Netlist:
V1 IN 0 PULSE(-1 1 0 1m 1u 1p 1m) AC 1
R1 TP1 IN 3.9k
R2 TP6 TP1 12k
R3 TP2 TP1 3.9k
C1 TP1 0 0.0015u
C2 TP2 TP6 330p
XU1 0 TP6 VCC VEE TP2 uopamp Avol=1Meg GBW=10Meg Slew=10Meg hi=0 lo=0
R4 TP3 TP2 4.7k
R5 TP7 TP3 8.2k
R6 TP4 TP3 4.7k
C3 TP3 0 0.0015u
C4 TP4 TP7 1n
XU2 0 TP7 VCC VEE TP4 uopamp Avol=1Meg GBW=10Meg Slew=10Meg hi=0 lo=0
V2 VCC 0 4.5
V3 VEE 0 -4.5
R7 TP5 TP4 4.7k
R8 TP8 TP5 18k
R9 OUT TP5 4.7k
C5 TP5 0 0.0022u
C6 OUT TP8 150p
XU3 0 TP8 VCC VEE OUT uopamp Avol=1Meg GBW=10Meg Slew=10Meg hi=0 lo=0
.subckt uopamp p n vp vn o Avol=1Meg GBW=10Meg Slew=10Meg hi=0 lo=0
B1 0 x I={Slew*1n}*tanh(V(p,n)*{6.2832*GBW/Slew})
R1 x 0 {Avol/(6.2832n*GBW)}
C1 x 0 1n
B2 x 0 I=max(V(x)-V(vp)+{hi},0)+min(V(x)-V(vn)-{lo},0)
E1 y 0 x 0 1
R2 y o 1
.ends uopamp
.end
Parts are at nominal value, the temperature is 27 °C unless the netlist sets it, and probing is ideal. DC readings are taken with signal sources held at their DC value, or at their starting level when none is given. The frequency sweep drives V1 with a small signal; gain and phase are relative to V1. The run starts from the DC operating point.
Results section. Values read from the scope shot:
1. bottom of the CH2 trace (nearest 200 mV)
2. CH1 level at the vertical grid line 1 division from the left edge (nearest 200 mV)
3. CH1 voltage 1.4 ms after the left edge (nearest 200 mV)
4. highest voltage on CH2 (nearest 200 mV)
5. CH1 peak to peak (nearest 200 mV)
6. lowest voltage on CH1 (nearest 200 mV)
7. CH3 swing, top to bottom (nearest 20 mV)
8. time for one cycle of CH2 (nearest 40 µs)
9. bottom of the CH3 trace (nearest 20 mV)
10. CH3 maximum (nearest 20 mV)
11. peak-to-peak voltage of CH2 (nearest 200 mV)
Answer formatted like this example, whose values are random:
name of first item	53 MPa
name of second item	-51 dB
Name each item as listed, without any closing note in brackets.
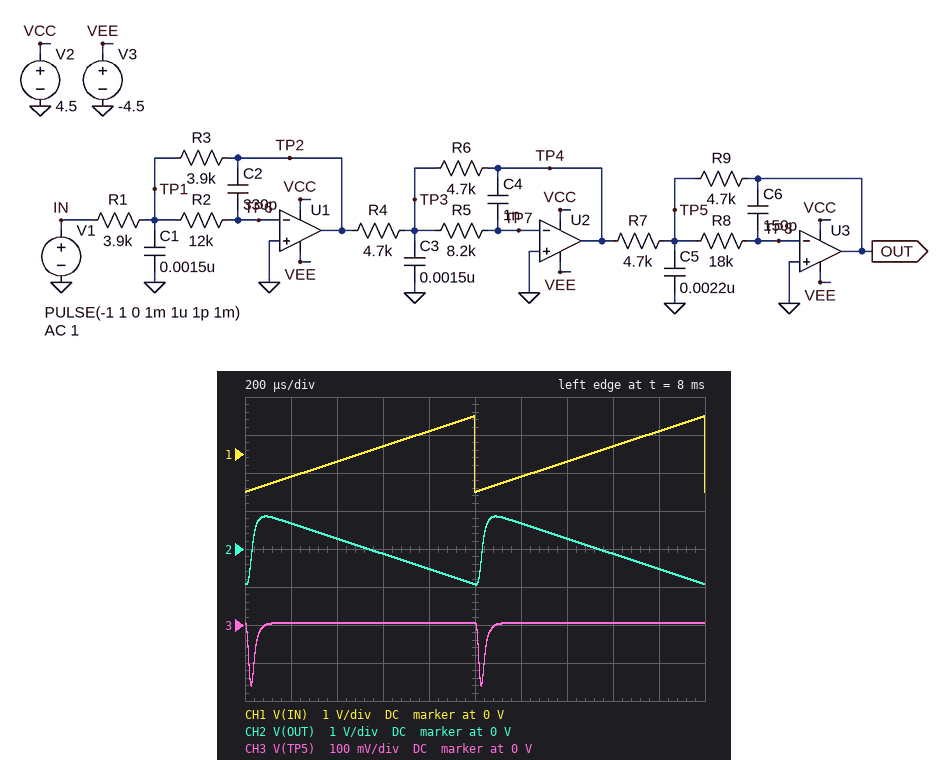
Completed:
bottom of the CH2 trace	-1.0 V
CH1 level at the vertical grid line 1 division from the left edge	-600 mV
CH1 voltage 1.4 ms after the left edge	-200 mV
highest voltage on CH2	800 mV
CH1 peak to peak	2.0 V
lowest voltage on CH1	-1.0 V
CH3 swing, top to bottom	160 mV
time for one cycle of CH2	1.00 ms
bottom of the CH3 trace	-160 mV
CH3 maximum	0 V
peak-to-peak voltage of CH2	1.8 V
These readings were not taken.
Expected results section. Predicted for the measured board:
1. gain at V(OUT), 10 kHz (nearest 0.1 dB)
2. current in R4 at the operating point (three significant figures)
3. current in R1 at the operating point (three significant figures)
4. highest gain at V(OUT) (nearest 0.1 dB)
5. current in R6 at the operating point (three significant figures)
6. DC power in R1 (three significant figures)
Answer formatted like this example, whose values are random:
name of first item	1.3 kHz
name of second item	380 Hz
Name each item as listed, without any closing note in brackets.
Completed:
gain at V(OUT), 10 kHz	-4.1 dB
current in R4 at the operating point	213 µA
current in R1 at the operating point	256 µA
highest gain at V(OUT)	0 dB
current in R6 at the operating point	213 µA
DC power in R1	256 µW
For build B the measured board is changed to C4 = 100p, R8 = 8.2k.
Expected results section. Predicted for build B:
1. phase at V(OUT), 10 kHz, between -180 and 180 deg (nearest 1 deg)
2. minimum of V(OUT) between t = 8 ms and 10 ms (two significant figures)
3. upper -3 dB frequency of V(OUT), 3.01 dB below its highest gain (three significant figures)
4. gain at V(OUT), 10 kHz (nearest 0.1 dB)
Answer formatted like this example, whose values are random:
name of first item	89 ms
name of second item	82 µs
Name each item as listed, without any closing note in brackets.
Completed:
phase at V(OUT), 10 kHz, between -180 and 180 deg	128 deg
minimum of V(OUT) between t = 8 ms and 10 ms	-980 mV
upper -3 dB frequency of V(OUT), 3.01 dB below its highest gain	36.0 kHz
gain at V(OUT), 10 kHz	-0.3 dB
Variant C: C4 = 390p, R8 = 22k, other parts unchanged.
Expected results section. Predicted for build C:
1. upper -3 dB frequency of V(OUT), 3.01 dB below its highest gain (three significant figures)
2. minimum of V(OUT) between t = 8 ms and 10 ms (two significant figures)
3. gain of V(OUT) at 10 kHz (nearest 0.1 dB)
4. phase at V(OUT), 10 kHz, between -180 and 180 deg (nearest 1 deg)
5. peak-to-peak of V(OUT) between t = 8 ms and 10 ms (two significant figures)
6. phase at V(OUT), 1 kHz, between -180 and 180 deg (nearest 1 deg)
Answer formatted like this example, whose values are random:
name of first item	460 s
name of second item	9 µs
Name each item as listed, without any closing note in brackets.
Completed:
upper -3 dB frequency of V(OUT), 3.01 dB below its highest gain	17.2 kHz
minimum of V(OUT) between t = 8 ms and 10 ms	-960 mV
gain of V(OUT) at 10 kHz	-0.9 dB
phase at V(OUT), 10 kHz, between -180 and 180 deg	90 deg
peak-to-peak of V(OUT) between t = 8 ms and 10 ms	2.0 V
phase at V(OUT), 1 kHz, between -180 and 180 deg	171 deg
